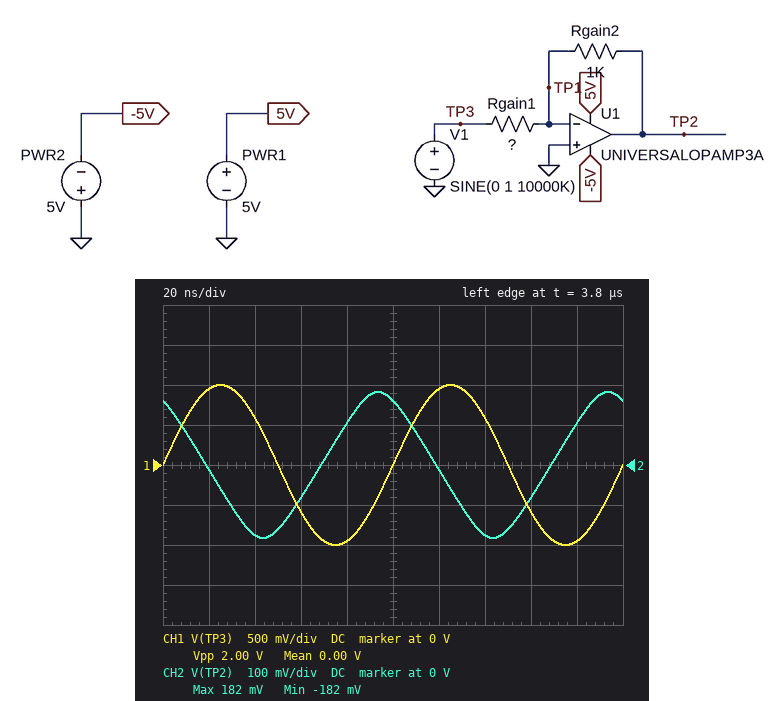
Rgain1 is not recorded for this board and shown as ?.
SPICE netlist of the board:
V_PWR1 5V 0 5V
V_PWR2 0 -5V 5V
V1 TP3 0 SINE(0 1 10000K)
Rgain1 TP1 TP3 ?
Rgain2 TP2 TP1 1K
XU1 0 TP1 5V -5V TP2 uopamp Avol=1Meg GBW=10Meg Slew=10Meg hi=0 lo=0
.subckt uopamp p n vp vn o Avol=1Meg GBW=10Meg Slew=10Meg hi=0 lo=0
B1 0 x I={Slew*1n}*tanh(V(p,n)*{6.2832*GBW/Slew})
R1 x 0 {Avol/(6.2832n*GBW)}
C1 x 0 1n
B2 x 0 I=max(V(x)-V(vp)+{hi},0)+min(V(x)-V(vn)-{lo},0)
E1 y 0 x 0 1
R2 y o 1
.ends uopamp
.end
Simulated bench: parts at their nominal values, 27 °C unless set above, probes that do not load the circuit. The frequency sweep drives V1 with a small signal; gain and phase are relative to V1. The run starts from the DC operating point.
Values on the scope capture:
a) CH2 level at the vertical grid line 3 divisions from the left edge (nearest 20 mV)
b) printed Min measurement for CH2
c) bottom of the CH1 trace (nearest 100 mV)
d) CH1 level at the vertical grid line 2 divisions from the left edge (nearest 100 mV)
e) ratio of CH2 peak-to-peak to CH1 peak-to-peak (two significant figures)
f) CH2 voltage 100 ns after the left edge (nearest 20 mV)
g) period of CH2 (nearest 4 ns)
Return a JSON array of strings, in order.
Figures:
["-80 mV", "-182 mV", "-1.0 V", "600 mV", "0.18", "160 mV", "100 ns"]
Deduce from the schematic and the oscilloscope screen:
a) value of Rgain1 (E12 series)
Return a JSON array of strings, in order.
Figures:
["2.2 kΩ"]
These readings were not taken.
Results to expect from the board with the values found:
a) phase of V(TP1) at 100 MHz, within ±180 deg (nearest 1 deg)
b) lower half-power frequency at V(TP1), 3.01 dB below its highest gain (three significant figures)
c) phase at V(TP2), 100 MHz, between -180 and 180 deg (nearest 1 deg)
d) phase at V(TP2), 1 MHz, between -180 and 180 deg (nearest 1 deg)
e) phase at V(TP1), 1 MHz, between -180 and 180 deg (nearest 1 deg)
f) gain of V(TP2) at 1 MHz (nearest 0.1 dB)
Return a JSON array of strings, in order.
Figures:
["4 deg", "6.87 MHz", "93 deg", "172 deg", "82 deg", "-6.9 dB"]
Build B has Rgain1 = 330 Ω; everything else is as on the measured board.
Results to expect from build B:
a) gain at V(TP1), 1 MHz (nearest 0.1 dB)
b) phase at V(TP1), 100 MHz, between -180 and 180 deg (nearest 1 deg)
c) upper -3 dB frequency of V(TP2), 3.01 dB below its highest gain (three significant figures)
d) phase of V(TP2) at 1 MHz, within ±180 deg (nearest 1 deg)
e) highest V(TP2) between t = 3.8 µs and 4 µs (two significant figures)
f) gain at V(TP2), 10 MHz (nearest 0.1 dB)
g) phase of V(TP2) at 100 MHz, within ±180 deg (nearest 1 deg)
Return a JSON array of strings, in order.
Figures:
["-11.0 dB", "1 deg", "2.48 MHz", "158 deg", "230 mV", "-2.7 dB", "91 deg"]
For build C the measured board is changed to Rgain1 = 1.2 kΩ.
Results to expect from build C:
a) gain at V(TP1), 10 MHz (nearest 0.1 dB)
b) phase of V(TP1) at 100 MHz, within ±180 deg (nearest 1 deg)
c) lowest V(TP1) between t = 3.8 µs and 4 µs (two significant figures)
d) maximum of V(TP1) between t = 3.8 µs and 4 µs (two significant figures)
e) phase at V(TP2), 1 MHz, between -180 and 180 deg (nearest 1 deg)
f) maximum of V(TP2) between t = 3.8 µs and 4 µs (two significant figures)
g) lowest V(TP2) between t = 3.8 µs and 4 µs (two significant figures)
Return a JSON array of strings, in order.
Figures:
["-8.0 dB", "3 deg", "-440 mV", "440 mV", "170 deg", "210 mV", "-210 mV"]
